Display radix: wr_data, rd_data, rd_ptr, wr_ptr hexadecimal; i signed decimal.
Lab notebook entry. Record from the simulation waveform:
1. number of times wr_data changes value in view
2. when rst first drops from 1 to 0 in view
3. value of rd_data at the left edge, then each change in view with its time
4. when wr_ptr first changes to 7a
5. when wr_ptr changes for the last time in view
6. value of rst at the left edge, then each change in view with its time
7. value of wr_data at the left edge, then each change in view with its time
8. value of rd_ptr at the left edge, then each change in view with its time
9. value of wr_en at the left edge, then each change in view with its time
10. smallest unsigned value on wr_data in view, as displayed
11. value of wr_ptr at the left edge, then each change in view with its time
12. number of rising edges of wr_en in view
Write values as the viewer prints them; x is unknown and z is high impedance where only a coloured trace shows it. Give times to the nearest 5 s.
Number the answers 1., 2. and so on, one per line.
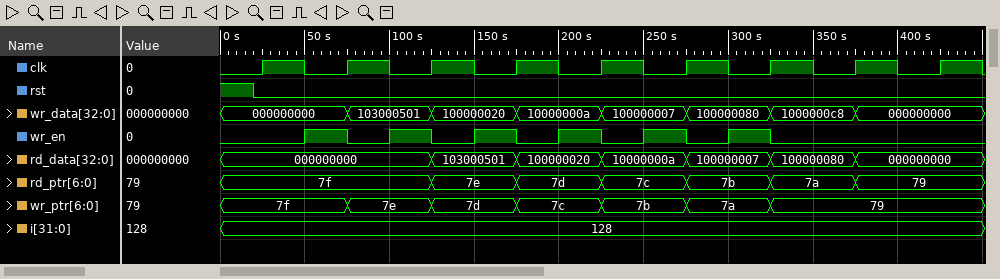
1. 7
2. 20 s
3. 000000000, 103000501 at 125 s, 100000020 at 175 s, 10000000a at 225 s, 100000007 at 275 s, 100000080 at 325 s, 000000000 at 375 s
4. 275 s
5. 325 s
6. 1, 0 at 20 s
7. 000000000, 103000501 at 75 s, 100000020 at 125 s, 10000000a at 175 s, 100000007 at 225 s, 100000080 at 275 s, 1000000c8 at 325 s, 000000000 at 375 s
8. 7f, 7e at 125 s, 7d at 175 s, 7c at 225 s, 7b at 275 s, 7a at 325 s, 79 at 375 s
9. 0, 1 at 50 s, 0 at 75 s, 1 at 100 s, 0 at 125 s, 1 at 150 s, 0 at 175 s, 1 at 200 s, 0 at 225 s, 1 at 250 s, 0 at 275 s, 1 at 300 s, 0 at 325 s
10. 000000000
11. 7f, 7e at 75 s, 7d at 125 s, 7c at 175 s, 7b at 225 s, 7a at 275 s, 79 at 325 s
12. 6
